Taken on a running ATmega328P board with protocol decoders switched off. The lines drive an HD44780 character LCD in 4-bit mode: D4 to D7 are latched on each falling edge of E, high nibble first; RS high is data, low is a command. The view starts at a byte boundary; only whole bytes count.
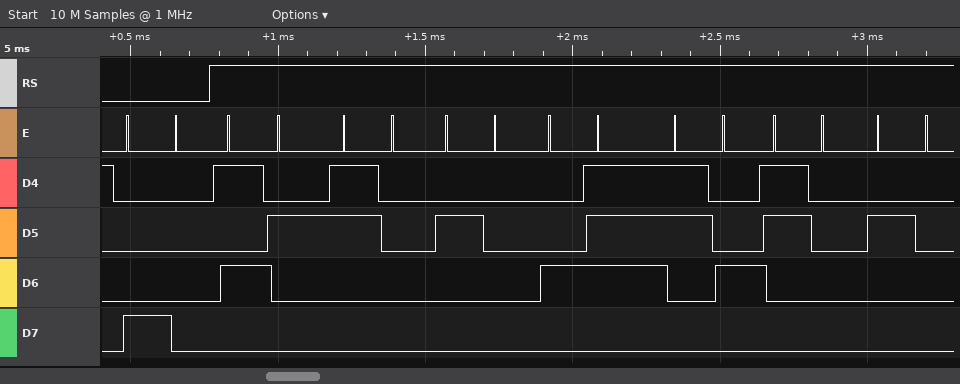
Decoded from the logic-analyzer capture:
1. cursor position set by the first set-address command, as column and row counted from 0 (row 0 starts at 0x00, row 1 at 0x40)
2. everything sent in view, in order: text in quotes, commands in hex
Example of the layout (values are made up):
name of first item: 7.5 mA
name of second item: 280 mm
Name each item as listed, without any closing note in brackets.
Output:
cursor position set by the first set-address command, as column and row counted from 0: column 0, row 0
everything sent in view, in order: text in quotes, commands in hex: 0x80 "R0 G40 "
